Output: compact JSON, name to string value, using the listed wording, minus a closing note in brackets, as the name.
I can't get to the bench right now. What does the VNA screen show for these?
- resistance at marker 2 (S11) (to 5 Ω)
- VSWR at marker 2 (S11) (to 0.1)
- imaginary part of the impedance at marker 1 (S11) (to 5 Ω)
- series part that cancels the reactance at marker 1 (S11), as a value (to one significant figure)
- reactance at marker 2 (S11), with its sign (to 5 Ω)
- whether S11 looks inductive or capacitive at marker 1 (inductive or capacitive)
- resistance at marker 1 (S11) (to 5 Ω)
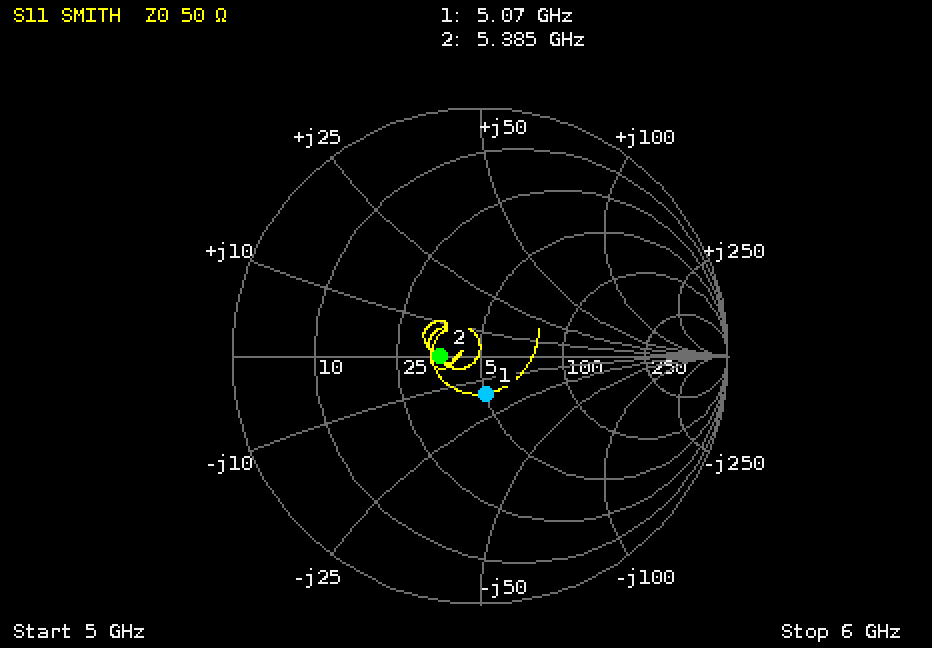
{"resistance at marker 2 (S11)": "35 Ω", "VSWR at marker 2 (S11)": "1.4", "imaginary part of the impedance at marker 1 (S11)": "-15 Ω", "series part that cancels the reactance at marker 1 (S11), as a value": "500 pH", "reactance at marker 2 (S11), with its sign": "0 Ω", "whether S11 looks inductive or capacitive at marker 1": "capacitive", "resistance at marker 1 (S11)": "50 Ω"}
